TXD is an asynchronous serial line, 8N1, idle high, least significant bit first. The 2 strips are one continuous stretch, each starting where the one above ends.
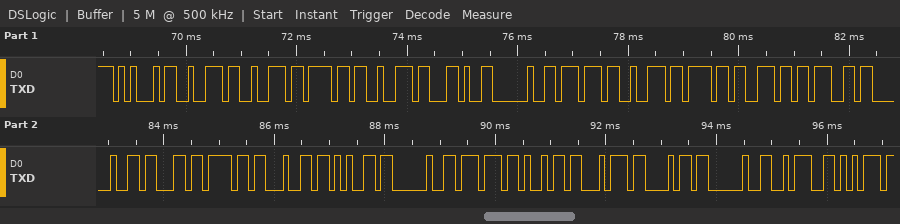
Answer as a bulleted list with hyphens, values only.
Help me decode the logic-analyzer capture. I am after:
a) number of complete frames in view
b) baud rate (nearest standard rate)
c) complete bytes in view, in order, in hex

- 25
- 9600 baud
- 45 72 72 6F 72 2C 20 77 72 6F 6E 67 20 63 6F 64 65 20 77 69 74 68 20 3A 75
